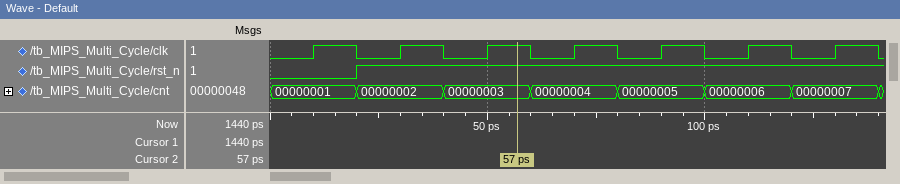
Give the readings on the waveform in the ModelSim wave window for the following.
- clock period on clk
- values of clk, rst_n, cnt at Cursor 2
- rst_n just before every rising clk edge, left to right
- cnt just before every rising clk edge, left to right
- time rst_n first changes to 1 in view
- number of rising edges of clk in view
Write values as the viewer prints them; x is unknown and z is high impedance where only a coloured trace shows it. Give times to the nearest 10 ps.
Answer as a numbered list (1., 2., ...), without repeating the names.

1. 20 ps
2. clk=1, rst_n=1, cnt=00000003
3. 0 1 1 1 1 1 1
4. 00000001, 00000002, 00000003, 00000004, 00000005, 00000006, 00000007
5. 20 ps
6. 7
